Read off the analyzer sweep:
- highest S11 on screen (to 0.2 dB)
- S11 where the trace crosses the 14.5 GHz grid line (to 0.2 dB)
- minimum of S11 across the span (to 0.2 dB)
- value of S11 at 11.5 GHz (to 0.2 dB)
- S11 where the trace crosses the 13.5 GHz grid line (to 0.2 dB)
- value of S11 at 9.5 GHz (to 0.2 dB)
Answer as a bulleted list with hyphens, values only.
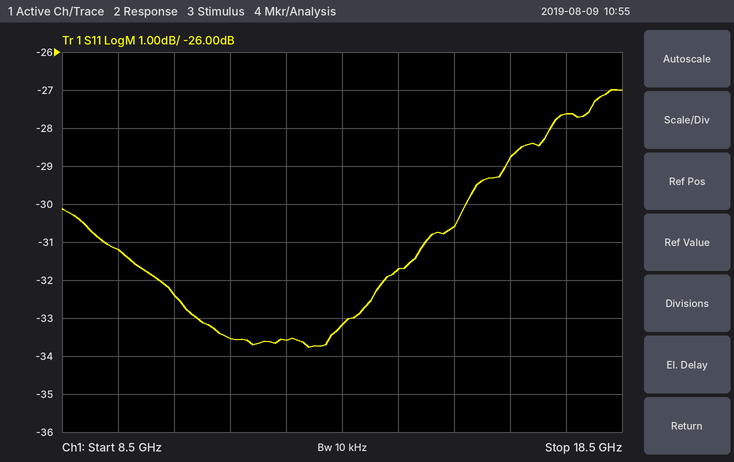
- -27.0 dB
- -31.8 dB
- -33.8 dB
- -33.6 dB
- -33.2 dB
- -31.2 dB
